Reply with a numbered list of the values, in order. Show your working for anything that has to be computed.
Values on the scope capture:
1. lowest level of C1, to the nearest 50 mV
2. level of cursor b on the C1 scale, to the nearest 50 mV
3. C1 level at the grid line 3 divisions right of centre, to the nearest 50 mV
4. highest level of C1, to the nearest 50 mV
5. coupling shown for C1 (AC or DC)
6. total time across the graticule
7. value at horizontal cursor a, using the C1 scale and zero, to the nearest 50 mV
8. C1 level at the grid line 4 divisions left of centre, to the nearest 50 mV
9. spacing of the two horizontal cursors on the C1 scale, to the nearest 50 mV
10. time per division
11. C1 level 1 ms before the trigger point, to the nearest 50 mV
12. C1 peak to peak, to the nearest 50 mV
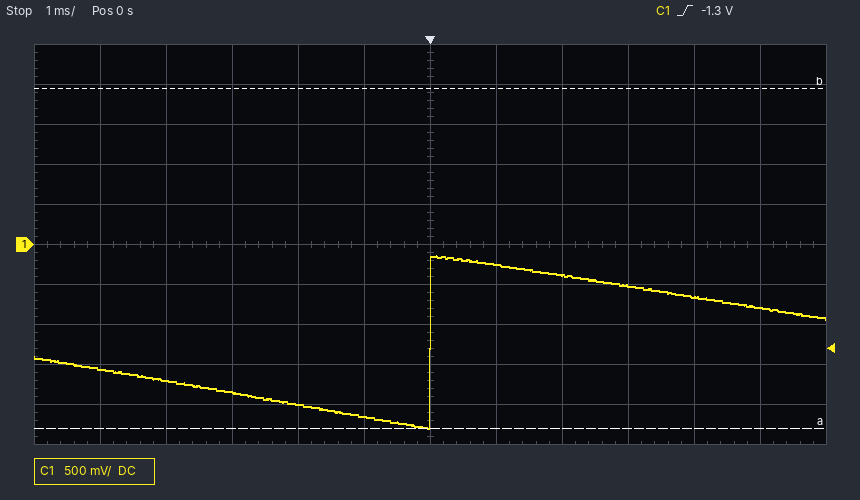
1. -2.30 V
2. 1.95 V
3. -500 mV
4. -150 mV
5. DC
6. 12 ms
7. -2.30 V
8. -1.70 V
9. 4.25 V
10. 1 ms
11. -2.15 V
12. -150 mV − (-2.30 V) = 2.15 V
